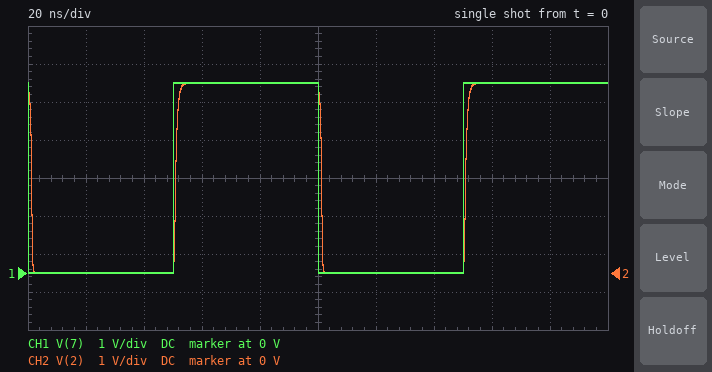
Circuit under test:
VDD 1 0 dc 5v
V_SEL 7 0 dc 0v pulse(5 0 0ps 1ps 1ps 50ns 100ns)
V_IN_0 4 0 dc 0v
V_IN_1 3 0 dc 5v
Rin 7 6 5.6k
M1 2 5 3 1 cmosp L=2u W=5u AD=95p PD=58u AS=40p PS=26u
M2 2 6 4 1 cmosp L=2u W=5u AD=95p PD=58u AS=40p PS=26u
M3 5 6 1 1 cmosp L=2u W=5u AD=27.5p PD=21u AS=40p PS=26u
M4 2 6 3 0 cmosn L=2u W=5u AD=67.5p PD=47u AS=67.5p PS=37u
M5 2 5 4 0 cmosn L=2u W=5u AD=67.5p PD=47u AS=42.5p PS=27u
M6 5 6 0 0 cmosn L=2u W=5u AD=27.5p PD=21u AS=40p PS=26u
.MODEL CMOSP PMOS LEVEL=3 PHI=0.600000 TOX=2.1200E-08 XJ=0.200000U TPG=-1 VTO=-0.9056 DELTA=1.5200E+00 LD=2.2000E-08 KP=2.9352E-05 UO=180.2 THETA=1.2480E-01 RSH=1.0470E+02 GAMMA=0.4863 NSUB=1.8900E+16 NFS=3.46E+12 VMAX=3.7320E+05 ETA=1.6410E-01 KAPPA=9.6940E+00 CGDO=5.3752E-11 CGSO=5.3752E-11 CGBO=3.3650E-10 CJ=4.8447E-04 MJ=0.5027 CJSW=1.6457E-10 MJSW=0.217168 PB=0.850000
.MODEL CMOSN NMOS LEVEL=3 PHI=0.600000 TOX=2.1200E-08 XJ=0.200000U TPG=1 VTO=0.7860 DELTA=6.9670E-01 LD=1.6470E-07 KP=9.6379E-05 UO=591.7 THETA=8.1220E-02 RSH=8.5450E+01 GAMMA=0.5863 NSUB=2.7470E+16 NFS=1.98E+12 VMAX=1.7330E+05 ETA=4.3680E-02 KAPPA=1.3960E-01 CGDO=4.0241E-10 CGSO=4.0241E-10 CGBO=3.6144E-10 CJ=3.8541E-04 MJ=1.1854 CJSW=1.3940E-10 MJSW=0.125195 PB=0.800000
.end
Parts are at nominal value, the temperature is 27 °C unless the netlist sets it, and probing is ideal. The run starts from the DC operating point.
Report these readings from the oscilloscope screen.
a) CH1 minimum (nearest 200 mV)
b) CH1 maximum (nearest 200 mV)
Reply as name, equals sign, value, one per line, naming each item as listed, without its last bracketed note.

CH1 minimum = 0 V
CH1 maximum = 5.0 V
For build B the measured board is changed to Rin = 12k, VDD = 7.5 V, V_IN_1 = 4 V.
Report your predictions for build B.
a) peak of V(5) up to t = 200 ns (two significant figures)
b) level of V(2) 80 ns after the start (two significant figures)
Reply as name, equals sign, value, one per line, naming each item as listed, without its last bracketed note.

peak of V(5) up to t = 200 ns = 7.6 V
level of V(2) 80 ns after the start = 4.0 V
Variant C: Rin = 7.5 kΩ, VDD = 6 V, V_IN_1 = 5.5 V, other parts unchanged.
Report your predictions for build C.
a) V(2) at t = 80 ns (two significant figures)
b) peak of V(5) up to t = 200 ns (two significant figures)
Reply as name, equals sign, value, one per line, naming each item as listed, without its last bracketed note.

V(2) at t = 80 ns = 5.5 V
peak of V(5) up to t = 200 ns = 6.2 V
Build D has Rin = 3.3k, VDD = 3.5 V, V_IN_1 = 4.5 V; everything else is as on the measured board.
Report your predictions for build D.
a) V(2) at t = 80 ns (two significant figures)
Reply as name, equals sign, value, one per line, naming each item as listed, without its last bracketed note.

V(2) at t = 80 ns = 4.0 V
